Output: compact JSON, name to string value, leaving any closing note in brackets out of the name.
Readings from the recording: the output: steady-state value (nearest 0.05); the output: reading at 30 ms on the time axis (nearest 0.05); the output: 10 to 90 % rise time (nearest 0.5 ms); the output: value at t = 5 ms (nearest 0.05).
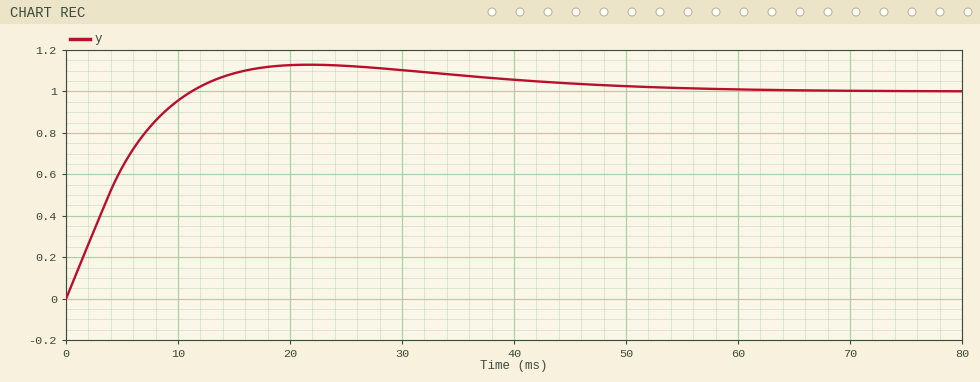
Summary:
{"the output: steady-state value": "1.00", "the output: reading at 30 ms on the time axis": "1.10", "the output: 10 to 90 % rise time": "8.0 ms", "the output: value at t = 5 ms": "0.65"}
